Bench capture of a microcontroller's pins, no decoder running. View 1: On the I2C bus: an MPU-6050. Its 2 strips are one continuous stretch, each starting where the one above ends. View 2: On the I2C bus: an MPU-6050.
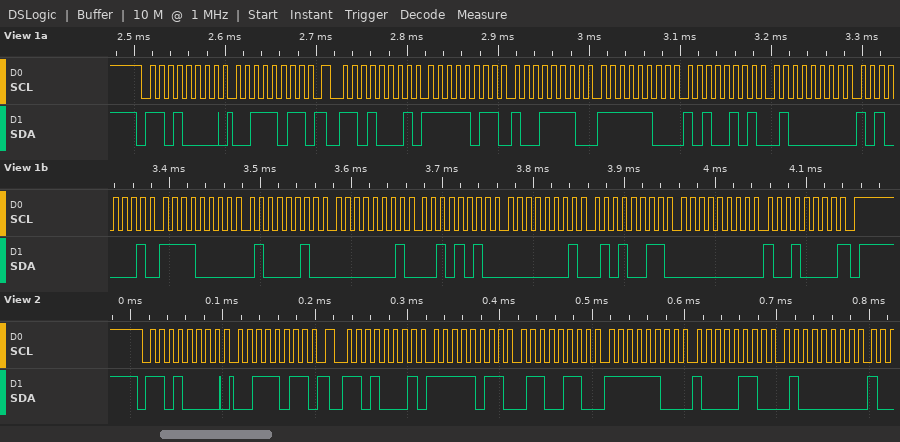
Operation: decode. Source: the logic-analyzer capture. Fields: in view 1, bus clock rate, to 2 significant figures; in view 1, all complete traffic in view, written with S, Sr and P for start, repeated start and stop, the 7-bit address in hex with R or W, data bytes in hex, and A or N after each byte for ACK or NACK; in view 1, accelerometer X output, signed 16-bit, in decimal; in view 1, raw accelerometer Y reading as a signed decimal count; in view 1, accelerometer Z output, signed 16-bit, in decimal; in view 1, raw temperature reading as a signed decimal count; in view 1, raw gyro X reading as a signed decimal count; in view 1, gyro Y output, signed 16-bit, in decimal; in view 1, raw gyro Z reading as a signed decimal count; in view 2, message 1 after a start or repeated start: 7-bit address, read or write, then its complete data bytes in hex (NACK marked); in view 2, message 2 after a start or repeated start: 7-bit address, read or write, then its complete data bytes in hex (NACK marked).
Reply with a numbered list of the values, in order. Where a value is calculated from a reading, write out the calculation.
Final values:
1. 100 kHz
2. S 68W A 3B A Sr 68R A FB A 9E A FC A A5 A 40 A A1 A F0 A 42 A 01 A 2A A 01 A 53 A 00 A 90 N P
3. 0xFB9E = -1122
4. 0xFCA5 = -859
5. 0x40A1 = 16545
6. 0xF042 = -4030
7. 0x012A = 298
8. 0x0153 = 339
9. 0x0090 = 144
10. 0x68 write: 3B
11. 0x68 read: FB 66 FC 86 40
